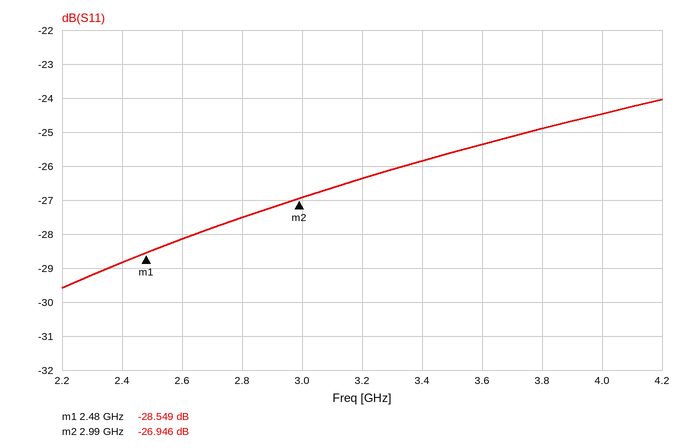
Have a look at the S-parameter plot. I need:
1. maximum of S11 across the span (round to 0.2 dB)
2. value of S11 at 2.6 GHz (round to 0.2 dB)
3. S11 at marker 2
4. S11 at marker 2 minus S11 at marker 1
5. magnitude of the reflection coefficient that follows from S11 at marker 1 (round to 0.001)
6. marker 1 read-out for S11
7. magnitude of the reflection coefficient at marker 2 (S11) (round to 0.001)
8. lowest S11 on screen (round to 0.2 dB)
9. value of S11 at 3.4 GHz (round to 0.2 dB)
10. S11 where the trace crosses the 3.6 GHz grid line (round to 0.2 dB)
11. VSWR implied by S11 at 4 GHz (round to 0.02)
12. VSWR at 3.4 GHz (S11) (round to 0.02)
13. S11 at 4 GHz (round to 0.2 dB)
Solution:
-24.0 dB
-28.2 dB
-26.946 dB
1.603 dB
0.037
-28.549 dB
0.045
-29.6 dB
-25.8 dB
-25.4 dB
1.12
1.10
-24.4 dB
